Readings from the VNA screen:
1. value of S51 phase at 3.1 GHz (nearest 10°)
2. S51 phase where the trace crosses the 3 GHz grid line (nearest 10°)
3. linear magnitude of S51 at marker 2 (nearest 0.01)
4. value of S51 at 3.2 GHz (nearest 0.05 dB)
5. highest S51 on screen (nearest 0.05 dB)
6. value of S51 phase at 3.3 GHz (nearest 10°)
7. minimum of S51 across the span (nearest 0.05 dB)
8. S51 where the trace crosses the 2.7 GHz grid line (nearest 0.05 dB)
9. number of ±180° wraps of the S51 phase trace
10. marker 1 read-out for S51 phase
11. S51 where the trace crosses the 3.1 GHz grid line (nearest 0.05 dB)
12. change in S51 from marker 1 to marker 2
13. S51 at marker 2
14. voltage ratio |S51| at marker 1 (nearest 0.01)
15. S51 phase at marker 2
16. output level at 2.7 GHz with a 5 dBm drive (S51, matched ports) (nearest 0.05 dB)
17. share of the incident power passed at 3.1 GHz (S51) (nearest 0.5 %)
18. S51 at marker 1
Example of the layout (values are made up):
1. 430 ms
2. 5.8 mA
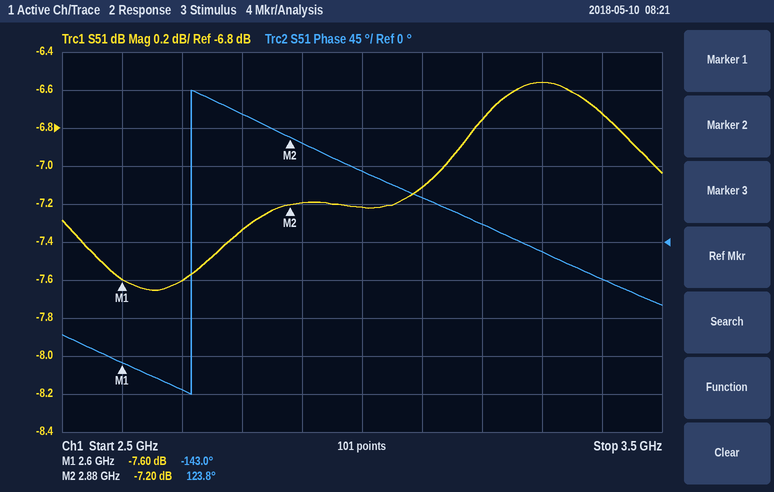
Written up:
1. 50°
2. 80°
3. 0.44
4. -6.75 dB
5. -6.55 dB
6. -10°
7. -7.65 dB
8. -7.60 dB
9. 1
10. -143.0°
11. -7.10 dB
12. 0.40 dB
13. -7.20 dB
14. 0.42
15. 123.8°
16. -2.60 dBm
17. 19.5 %
18. -7.60 dB
